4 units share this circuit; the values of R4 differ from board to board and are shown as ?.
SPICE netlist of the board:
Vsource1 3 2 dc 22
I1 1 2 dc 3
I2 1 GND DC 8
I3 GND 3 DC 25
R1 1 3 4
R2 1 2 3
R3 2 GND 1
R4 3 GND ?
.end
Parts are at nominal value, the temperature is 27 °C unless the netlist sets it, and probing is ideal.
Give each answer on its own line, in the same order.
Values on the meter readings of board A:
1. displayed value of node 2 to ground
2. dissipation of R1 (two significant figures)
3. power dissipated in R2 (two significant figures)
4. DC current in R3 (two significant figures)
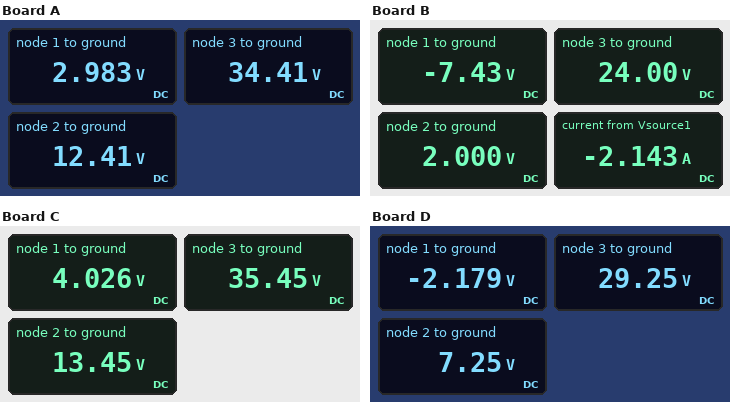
12.41 V
250 W
30 W
12 A
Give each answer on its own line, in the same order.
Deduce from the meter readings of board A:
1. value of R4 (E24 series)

7.5 Ω
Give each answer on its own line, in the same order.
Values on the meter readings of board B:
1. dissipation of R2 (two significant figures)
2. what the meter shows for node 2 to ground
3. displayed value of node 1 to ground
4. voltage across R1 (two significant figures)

30 W
2.000 V
-7.43 V
31 V
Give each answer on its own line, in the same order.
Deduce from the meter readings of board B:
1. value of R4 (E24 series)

1.6 Ω
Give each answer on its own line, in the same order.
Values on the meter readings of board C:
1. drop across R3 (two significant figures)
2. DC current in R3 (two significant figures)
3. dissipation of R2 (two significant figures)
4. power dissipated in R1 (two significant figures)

13 V
13 A
30 W
250 W
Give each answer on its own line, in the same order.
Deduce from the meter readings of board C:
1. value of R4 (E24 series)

10 Ω
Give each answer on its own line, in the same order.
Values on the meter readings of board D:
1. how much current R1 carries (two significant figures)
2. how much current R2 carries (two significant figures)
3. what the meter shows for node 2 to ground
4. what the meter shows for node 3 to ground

7.9 A
3.1 A
7.25 V
29.25 V
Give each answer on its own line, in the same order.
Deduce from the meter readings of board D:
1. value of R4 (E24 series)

3 Ω
